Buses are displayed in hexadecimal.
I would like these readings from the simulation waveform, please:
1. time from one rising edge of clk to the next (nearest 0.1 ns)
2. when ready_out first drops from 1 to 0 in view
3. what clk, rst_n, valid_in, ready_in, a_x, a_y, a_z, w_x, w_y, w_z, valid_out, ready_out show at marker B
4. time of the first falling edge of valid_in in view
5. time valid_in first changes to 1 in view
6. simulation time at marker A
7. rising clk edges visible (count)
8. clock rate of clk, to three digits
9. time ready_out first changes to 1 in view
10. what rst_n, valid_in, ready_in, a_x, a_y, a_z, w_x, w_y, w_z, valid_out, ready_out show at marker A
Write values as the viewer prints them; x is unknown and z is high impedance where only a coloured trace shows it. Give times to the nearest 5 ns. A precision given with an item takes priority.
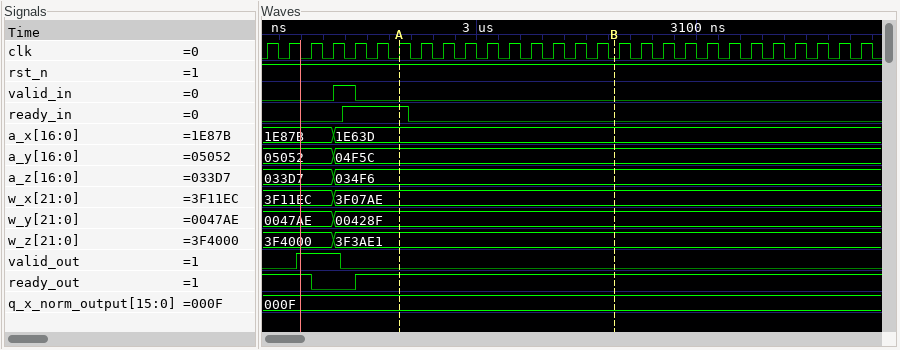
10 ns
2925 ns
clk=0, rst_n=1, valid_in=0, ready_in=0, a_x=1E63D, a_y=04F5C, a_z=034F6, w_x=3F07AE, w_y=00428F, w_z=3F3AE1, valid_out=0, ready_out=1
2945 ns
2935 ns
2965 ns
28
100 MHz
2945 ns
rst_n=1, valid_in=0, ready_in=1, a_x=1E63D, a_y=04F5C, a_z=034F6, w_x=3F07AE, w_y=00428F, w_z=3F3AE1, valid_out=0, ready_out=1
